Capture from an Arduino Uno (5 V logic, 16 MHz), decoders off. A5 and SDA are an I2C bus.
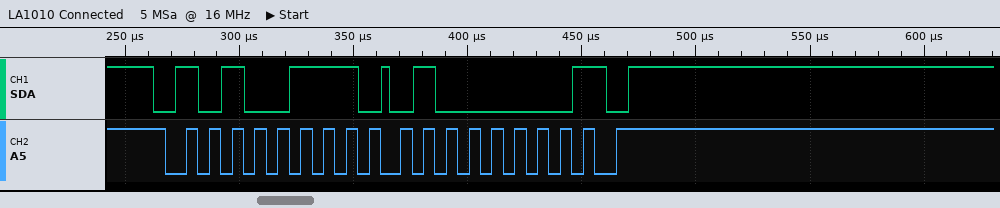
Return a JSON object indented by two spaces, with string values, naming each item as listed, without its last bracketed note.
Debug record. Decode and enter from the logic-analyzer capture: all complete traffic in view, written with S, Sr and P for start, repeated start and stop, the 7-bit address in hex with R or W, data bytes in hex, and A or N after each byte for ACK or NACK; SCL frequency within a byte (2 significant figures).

{
  "all complete traffic in view, written with S, Sr and P for start, repeated start and stop, the 7-bit address in hex with R or W, data bytes in hex, and A or N after each byte for ACK or NACK": "S 53R A 40 N P",
  "SCL frequency within a byte": "100 kHz"
}
